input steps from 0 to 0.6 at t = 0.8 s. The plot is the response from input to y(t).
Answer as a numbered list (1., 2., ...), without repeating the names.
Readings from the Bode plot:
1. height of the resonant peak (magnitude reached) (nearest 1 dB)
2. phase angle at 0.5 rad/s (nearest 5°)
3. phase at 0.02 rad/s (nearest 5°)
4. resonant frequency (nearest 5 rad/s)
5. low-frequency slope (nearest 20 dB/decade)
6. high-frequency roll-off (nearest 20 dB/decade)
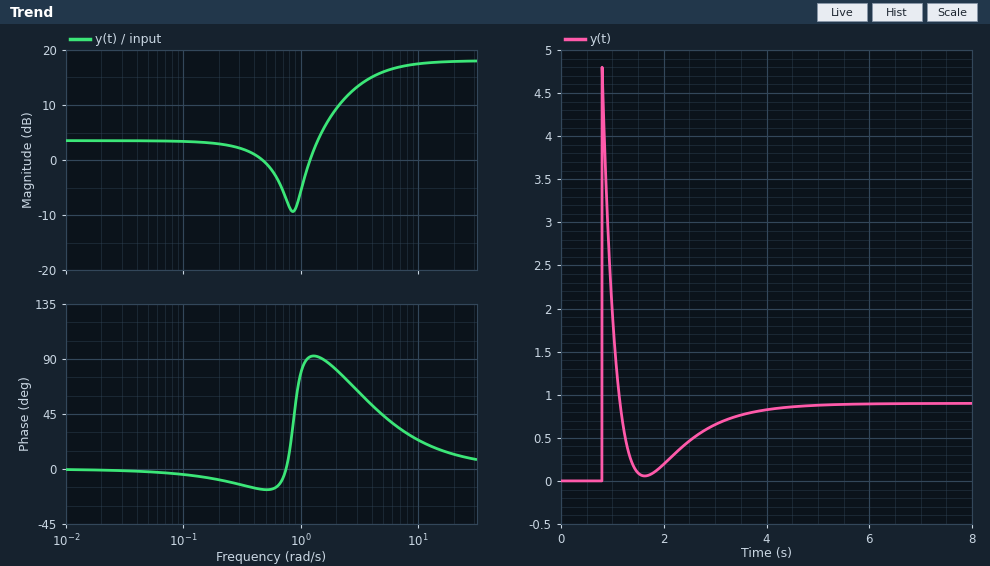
1. 18 dB
2. -15°
3. 0°
4. 20 rad/s
5. 0 dB/decade
6. 0 dB/decade
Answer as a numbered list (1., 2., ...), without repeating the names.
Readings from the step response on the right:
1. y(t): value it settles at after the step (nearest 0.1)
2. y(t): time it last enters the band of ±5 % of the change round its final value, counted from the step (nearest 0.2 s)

1. 0.9
2. 3.6 s
